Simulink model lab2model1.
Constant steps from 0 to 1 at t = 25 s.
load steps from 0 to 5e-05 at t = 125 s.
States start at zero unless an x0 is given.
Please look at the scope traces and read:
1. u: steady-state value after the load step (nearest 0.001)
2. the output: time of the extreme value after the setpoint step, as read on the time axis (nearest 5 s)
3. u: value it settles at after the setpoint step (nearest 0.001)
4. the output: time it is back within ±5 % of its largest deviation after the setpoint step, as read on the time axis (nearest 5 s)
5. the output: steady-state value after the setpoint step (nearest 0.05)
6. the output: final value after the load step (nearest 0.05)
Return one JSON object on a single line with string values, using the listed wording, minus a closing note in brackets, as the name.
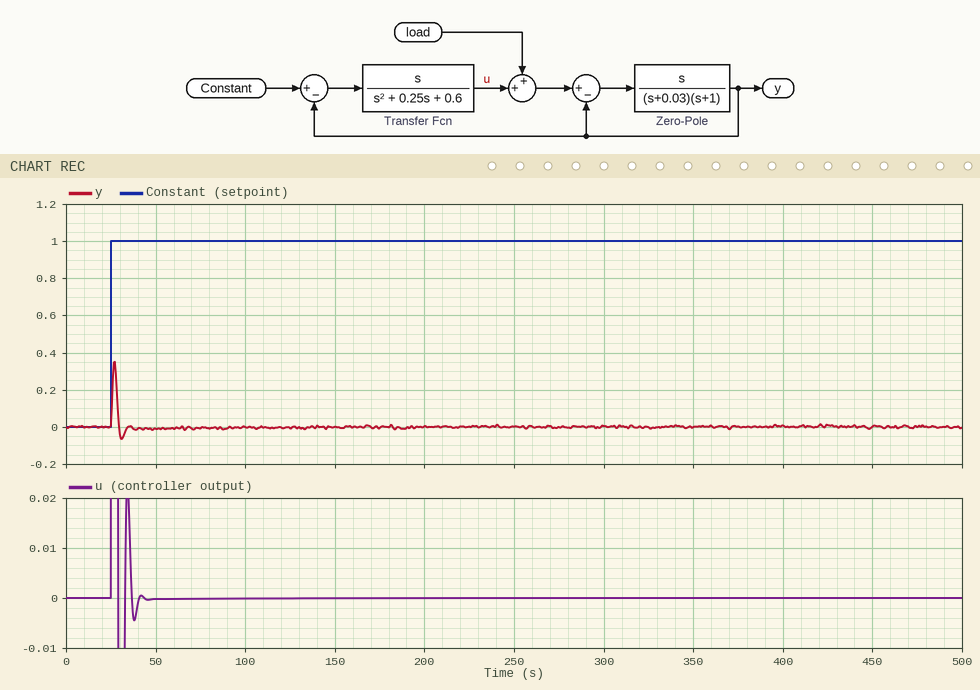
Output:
{"u: steady-state value after the load step": "0.000", "the output: time of the extreme value after the setpoint step, as read on the time axis": "25 s", "u: value it settles at after the setpoint step": "0.000", "the output: time it is back within ±5 % of its largest deviation after the setpoint step, as read on the time axis": "35 s", "the output: steady-state value after the setpoint step": "0.00", "the output: final value after the load step": "0.00"}
